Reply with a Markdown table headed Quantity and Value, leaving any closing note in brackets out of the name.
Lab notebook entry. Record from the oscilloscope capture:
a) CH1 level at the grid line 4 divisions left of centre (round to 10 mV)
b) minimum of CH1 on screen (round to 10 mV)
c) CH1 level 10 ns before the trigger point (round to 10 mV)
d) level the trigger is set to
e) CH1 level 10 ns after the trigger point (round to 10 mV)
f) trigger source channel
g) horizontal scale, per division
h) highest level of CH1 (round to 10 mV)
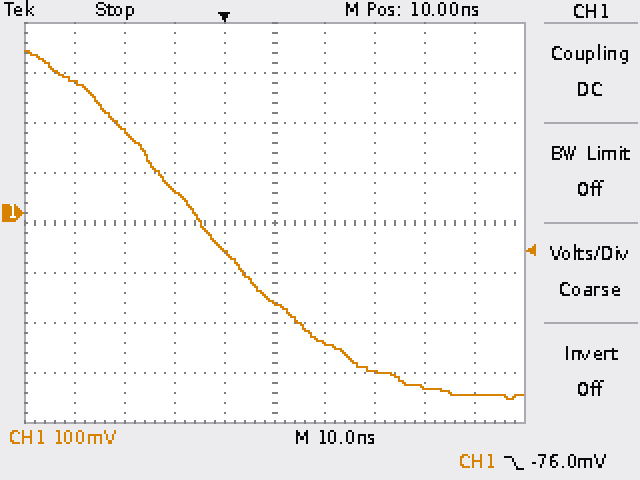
| Quantity | Value |
|---|---|
| CH1 level at the grid line 4 divisions left of centre | 260 mV |
| minimum of CH1 on screen | -370 mV |
| CH1 level 10 ns before the trigger point | 50 mV |
| level the trigger is set to | -76.0 mV |
| CH1 level 10 ns after the trigger point | -180 mV |
| trigger source channel | CH1 |
| horizontal scale, per division | 10 ns |
| highest level of CH1 | 320 mV |
